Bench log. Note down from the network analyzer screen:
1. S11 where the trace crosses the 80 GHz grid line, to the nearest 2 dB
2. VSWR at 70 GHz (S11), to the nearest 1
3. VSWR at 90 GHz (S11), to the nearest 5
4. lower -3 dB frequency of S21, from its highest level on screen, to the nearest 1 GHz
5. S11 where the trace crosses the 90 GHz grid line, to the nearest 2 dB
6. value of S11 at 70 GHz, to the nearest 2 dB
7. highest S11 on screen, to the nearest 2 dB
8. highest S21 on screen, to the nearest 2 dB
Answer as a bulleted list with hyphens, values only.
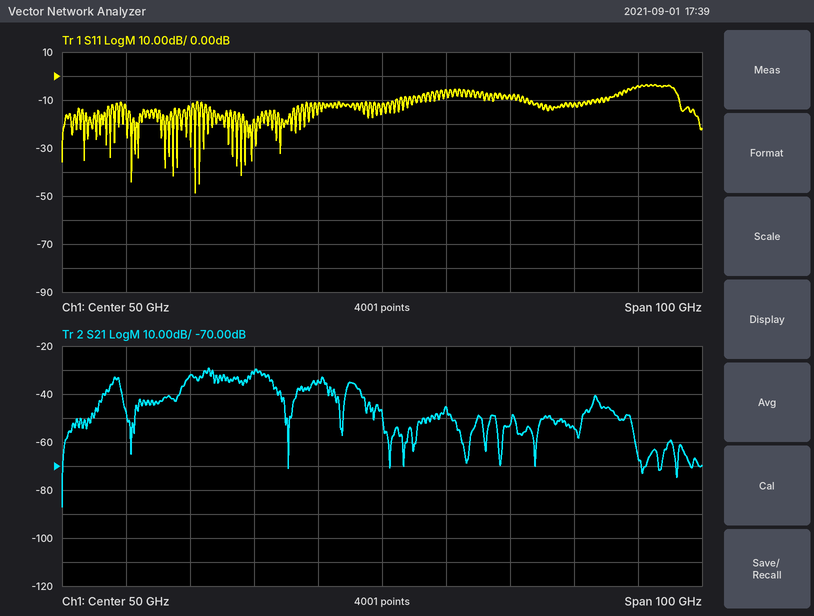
- -12 dB
- 2
- 5
- 22 GHz
- -4 dB
- -8 dB
- -4 dB
- -30 dB
